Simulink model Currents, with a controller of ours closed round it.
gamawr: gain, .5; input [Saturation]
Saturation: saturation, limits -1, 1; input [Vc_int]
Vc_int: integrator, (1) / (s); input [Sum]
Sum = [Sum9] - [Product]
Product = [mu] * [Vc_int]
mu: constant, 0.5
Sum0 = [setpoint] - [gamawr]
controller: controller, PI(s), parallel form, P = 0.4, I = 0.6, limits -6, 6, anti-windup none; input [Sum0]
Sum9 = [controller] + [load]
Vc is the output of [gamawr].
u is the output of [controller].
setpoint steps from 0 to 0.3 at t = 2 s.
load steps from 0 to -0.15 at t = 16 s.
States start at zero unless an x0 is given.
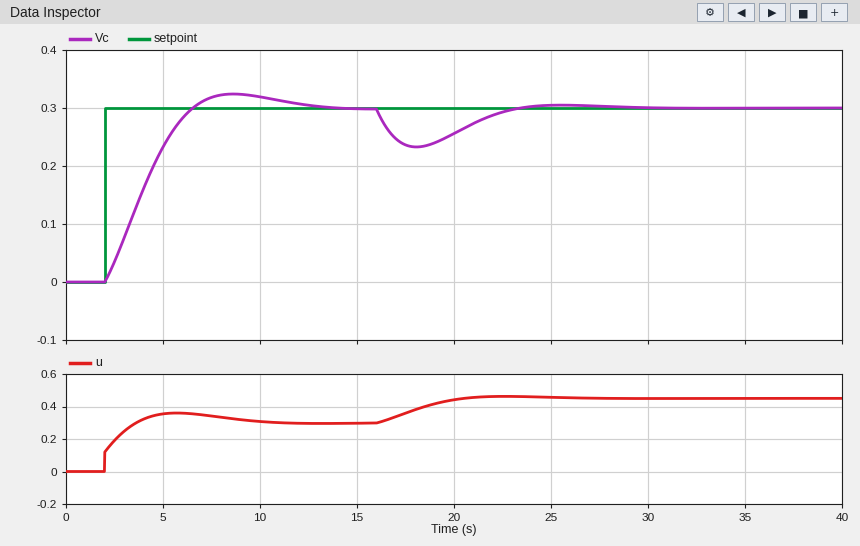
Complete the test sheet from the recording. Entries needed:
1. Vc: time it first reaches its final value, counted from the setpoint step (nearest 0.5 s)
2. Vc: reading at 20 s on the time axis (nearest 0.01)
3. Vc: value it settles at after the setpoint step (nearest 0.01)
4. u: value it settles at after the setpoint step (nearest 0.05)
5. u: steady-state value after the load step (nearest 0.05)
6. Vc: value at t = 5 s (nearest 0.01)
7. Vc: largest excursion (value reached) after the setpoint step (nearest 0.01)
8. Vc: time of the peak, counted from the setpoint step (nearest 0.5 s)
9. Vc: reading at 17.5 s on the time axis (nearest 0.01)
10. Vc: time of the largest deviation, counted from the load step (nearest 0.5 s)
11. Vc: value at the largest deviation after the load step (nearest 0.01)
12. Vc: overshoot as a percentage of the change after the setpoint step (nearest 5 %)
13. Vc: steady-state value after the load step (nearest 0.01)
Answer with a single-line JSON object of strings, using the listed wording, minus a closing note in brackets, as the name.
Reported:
{"Vc: time it first reaches its final value, counted from the setpoint step": "4.5 s", "Vc: reading at 20 s on the time axis": "0.26", "Vc: value it settles at after the setpoint step": "0.30", "u: value it settles at after the setpoint step": "0.30", "u: steady-state value after the load step": "0.45", "Vc: value at t = 5 s": "0.23", "Vc: largest excursion (value reached) after the setpoint step": "0.32", "Vc: time of the peak, counted from the setpoint step": "6.5 s", "Vc: reading at 17.5 s on the time axis": "0.24", "Vc: time of the largest deviation, counted from the load step": "2.0 s", "Vc: value at the largest deviation after the load step": "0.23", "Vc: overshoot as a percentage of the change after the setpoint step": "10 %", "Vc: steady-state value after the load step": "0.30"}
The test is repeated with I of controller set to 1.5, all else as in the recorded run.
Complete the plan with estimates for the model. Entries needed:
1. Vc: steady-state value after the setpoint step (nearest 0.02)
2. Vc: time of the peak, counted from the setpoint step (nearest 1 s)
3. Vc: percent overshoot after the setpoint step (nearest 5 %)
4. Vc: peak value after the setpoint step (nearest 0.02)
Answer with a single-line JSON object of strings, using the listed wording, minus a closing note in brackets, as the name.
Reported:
{"Vc: steady-state value after the setpoint step": "0.30", "Vc: time of the peak, counted from the setpoint step": "4 s", "Vc: percent overshoot after the setpoint step": "25 %", "Vc: peak value after the setpoint step": "0.38"}
